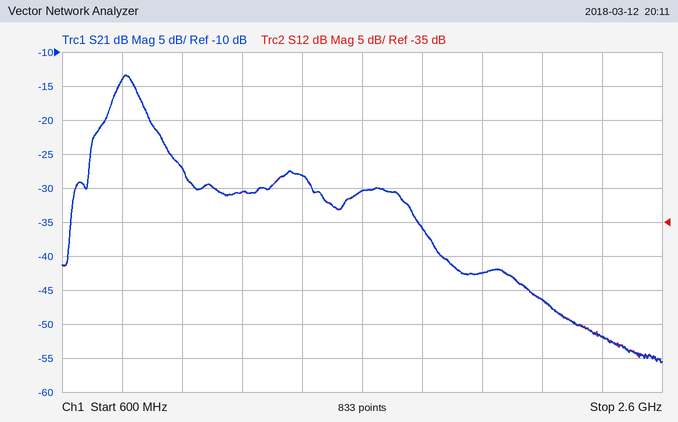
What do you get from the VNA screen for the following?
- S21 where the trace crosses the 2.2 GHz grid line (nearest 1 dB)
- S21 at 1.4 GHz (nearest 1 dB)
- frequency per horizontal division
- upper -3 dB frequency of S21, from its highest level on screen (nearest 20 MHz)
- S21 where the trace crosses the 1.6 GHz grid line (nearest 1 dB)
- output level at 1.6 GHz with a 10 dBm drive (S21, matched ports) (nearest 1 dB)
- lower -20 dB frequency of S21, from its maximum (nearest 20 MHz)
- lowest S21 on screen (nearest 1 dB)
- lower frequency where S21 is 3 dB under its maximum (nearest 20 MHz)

-46 dB
-28 dB
200 MHz
860 MHz
-30 dB
-20 dBm
640 MHz
-56 dB
780 MHz
